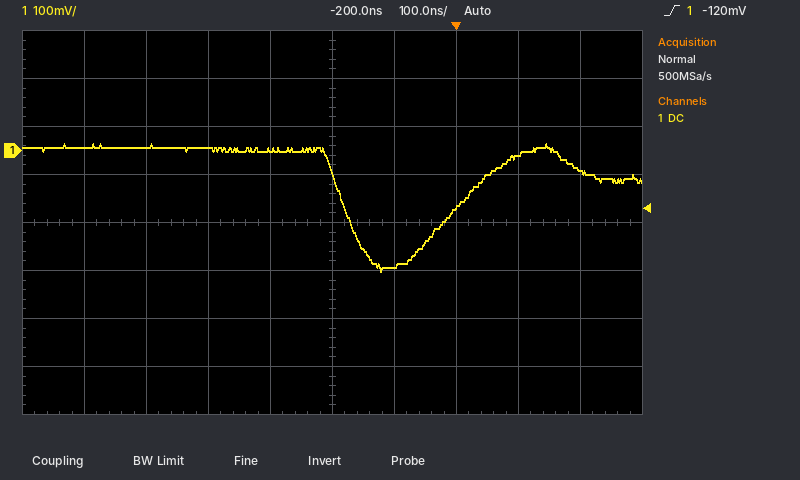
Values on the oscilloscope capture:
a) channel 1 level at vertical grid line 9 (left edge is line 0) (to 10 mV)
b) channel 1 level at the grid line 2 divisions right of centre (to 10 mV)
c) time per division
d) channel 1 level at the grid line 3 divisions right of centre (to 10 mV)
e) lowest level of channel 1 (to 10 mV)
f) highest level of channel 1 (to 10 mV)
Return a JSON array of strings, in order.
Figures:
["-40 mV", "-120 mV", "100 ns", "-10 mV", "-250 mV", "10 mV"]
